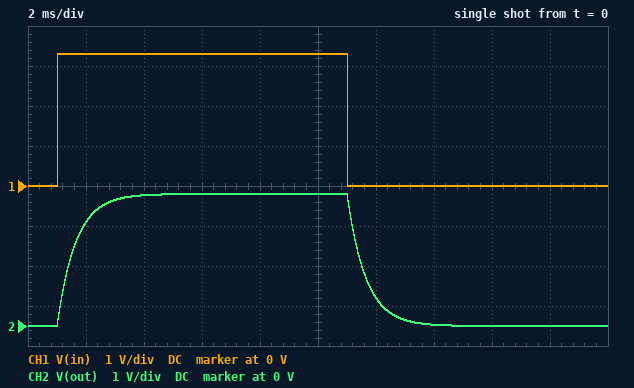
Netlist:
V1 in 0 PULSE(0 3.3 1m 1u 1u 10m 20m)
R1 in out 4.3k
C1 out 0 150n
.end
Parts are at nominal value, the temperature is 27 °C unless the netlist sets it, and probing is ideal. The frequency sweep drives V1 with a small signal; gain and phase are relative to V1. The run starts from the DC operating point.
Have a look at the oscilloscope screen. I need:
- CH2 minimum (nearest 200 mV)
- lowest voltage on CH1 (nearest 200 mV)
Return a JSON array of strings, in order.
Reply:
["0 V", "0 V"]
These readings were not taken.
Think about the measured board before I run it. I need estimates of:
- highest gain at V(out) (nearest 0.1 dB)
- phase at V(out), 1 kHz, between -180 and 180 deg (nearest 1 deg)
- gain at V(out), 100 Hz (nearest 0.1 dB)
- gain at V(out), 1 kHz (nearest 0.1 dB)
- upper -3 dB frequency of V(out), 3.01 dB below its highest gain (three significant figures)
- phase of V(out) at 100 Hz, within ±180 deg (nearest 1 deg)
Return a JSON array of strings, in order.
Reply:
["0 dB", "-76 deg", "-0.7 dB", "-12.4 dB", "247 Hz", "-22 deg"]
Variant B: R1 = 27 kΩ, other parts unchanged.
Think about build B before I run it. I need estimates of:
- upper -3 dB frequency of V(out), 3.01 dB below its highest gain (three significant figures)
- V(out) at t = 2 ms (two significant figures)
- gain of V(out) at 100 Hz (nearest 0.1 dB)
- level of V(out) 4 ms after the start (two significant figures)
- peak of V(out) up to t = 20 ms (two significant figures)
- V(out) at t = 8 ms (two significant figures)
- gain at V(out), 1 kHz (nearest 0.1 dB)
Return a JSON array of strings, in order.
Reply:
["39.3 Hz", "720 mV", "-8.7 dB", "1.7 V", "3.0 V", "2.7 V", "-28.1 dB"]
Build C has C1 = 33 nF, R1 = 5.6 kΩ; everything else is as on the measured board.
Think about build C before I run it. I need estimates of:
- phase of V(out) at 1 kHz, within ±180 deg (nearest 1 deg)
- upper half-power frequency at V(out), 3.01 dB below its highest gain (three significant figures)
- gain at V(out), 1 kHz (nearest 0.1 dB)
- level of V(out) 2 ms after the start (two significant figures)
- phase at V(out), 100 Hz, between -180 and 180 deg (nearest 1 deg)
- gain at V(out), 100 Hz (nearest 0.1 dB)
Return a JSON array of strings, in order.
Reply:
["-49 deg", "861 Hz", "-3.7 dB", "3.3 V", "-7 deg", "-0.1 dB"]
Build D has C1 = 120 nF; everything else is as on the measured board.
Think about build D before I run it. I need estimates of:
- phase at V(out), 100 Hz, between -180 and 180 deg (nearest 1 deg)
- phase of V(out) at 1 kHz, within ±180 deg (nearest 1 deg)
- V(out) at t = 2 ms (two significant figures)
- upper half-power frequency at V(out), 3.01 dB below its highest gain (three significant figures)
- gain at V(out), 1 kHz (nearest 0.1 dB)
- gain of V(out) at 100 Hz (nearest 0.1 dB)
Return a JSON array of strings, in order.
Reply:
["-18 deg", "-73 deg", "2.8 V", "308 Hz", "-10.6 dB", "-0.4 dB"]
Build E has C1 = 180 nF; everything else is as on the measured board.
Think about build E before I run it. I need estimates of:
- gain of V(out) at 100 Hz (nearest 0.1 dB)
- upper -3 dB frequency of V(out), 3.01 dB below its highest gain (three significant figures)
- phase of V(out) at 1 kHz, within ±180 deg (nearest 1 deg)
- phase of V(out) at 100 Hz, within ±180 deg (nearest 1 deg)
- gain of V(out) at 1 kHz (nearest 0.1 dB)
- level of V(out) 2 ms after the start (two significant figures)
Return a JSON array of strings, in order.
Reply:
["-0.9 dB", "206 Hz", "-78 deg", "-26 deg", "-13.9 dB", "2.4 V"]
